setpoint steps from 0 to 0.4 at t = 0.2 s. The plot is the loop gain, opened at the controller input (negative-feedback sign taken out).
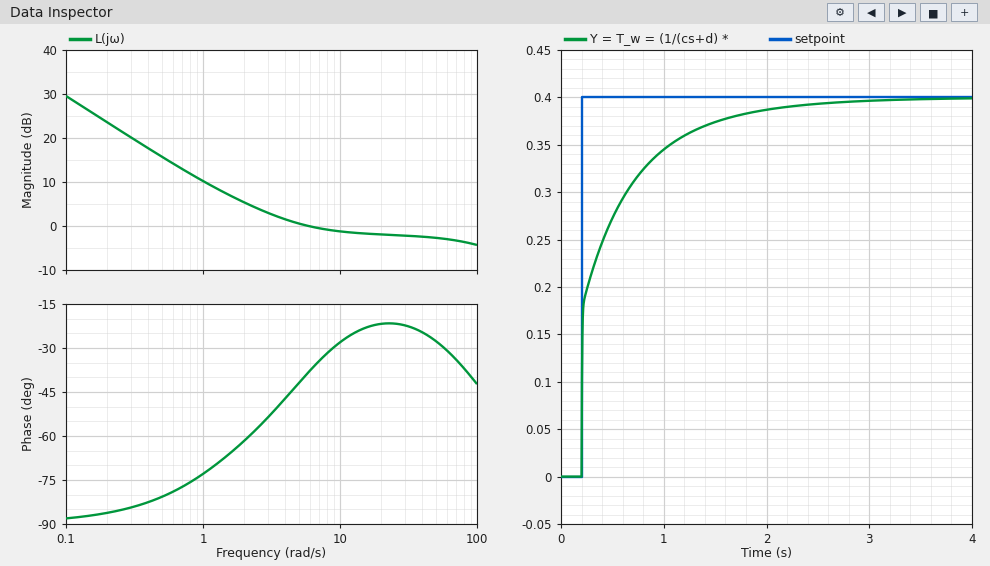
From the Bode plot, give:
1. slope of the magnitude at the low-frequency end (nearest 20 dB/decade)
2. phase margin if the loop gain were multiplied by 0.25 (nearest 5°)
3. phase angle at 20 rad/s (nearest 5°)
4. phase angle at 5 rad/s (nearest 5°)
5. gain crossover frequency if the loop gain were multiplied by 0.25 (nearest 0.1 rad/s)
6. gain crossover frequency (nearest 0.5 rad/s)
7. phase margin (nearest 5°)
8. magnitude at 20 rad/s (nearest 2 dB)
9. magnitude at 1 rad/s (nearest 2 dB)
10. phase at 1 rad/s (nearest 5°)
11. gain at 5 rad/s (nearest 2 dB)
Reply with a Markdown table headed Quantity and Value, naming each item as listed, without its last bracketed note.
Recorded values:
| Quantity | Value |
|---|---|
| slope of the magnitude at the low-frequency end | -20 dB/decade |
| phase margin if the loop gain were multiplied by 0.25 | 105° |
| phase angle at 20 rad/s | -20° |
| phase angle at 5 rad/s | -40° |
| gain crossover frequency if the loop gain were multiplied by 0.25 | 0.8 rad/s |
| gain crossover frequency | 6.0 rad/s |
| phase margin | 140° |
| magnitude at 20 rad/s | -2 dB |
| magnitude at 1 rad/s | 10 dB |
| phase at 1 rad/s | -75° |
| gain at 5 rad/s | 0 dB |
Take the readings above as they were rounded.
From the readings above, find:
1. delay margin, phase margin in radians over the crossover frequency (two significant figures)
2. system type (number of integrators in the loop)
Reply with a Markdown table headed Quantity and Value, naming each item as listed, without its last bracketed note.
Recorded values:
| Quantity | Value |
|---|---|
| delay margin, phase margin in radians over the crossover frequency | 0.41 s |
| system type | 1 |
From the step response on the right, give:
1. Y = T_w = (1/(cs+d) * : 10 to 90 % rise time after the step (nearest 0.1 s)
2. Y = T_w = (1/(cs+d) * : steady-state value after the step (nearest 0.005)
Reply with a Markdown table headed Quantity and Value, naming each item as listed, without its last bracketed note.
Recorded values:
| Quantity | Value |
|---|---|
| Y = T_w = (1/(cs+d) * : 10 to 90 % rise time after the step | 1.0 s |
| Y = T_w = (1/(cs+d) * : steady-state value after the step | 0.400 |
